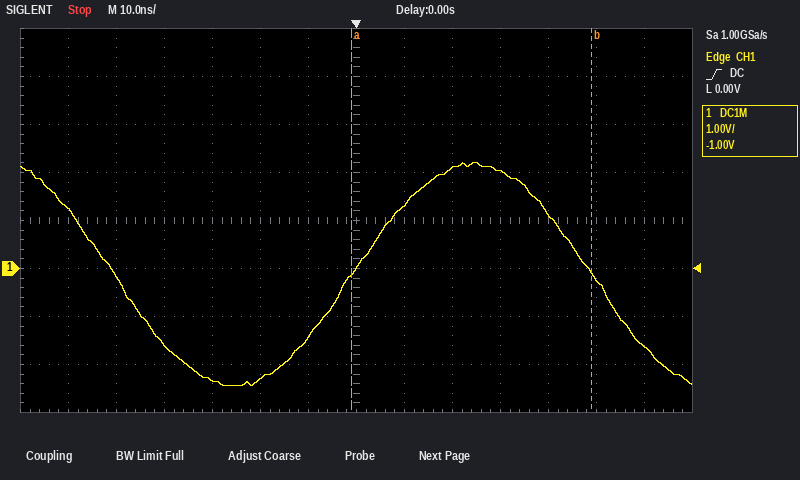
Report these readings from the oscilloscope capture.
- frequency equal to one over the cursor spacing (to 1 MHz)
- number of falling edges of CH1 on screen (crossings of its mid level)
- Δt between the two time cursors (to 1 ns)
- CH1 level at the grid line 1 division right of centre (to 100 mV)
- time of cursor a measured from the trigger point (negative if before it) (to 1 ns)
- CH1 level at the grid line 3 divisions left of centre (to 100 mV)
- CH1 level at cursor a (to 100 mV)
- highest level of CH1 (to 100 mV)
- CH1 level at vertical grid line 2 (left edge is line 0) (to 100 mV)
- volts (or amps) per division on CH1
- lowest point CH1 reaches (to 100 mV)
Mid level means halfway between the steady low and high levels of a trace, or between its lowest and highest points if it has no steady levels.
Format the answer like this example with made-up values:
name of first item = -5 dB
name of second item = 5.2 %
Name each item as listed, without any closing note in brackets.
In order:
frequency equal to one over the cursor spacing = 20 MHz
number of falling edges of CH1 on screen = 2
Δt between the two time cursors = 50 ns
CH1 level at the grid line 1 division right of centre = 1.3 V
time of cursor a measured from the trigger point (negative if before it) = -1 ns
CH1 level at the grid line 3 divisions left of centre = -2.3 V
CH1 level at cursor a = -100 mV
highest level of CH1 = 2.2 V
CH1 level at vertical grid line 2 (left edge is line 0) = -200 mV
volts (or amps) per division on CH1 = 1 V
lowest point CH1 reaches = -2.4 V
